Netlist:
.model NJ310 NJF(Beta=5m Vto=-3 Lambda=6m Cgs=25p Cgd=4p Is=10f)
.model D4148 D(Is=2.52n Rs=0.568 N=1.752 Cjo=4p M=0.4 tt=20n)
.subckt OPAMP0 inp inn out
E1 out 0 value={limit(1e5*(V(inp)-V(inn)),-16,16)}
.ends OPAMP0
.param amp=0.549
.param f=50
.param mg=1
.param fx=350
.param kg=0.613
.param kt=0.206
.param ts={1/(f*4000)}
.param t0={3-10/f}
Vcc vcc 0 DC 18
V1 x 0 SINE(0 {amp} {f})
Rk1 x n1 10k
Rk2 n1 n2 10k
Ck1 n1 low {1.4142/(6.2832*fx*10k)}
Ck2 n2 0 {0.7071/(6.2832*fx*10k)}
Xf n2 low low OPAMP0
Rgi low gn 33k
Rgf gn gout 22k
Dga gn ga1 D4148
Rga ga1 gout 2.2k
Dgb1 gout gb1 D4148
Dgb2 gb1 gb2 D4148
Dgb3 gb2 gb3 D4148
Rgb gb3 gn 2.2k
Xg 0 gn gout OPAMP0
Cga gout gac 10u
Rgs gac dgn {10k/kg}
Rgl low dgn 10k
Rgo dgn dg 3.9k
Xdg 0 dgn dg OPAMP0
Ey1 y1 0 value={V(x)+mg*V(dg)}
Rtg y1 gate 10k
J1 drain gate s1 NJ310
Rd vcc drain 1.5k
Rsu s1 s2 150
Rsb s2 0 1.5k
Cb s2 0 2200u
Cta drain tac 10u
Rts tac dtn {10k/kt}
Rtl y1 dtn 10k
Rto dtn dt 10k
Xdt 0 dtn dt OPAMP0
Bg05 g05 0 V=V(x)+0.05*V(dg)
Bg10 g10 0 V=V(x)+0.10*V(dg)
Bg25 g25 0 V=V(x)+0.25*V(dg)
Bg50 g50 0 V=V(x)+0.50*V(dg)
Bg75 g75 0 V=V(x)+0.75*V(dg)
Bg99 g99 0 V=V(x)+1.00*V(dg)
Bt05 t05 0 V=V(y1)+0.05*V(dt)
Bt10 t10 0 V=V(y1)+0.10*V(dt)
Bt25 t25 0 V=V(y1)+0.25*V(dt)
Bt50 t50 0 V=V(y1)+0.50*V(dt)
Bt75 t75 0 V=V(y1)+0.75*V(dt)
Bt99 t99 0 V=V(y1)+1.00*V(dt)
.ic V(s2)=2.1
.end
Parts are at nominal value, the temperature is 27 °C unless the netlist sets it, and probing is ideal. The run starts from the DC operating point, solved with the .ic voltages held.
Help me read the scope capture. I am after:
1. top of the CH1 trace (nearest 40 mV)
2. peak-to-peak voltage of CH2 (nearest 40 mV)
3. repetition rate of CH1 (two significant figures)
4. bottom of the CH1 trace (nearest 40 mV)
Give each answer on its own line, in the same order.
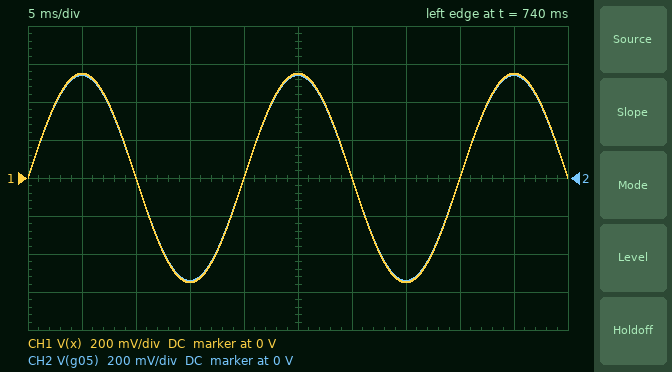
560 mV
1.08 V
50 Hz
-560 mV
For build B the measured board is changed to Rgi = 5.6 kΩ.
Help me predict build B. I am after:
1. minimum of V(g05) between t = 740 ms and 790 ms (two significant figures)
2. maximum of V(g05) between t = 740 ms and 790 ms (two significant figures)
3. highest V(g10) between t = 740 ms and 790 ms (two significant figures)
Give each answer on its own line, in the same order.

-550 mV
550 mV
550 mV
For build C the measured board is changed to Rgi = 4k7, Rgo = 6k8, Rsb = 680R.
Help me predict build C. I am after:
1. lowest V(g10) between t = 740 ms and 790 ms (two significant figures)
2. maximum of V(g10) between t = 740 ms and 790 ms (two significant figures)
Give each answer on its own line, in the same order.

-560 mV
550 mV
